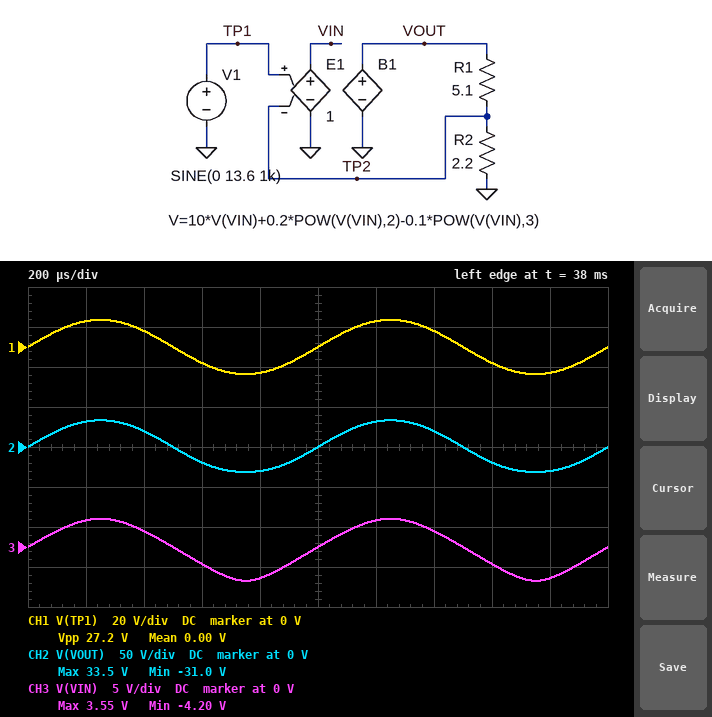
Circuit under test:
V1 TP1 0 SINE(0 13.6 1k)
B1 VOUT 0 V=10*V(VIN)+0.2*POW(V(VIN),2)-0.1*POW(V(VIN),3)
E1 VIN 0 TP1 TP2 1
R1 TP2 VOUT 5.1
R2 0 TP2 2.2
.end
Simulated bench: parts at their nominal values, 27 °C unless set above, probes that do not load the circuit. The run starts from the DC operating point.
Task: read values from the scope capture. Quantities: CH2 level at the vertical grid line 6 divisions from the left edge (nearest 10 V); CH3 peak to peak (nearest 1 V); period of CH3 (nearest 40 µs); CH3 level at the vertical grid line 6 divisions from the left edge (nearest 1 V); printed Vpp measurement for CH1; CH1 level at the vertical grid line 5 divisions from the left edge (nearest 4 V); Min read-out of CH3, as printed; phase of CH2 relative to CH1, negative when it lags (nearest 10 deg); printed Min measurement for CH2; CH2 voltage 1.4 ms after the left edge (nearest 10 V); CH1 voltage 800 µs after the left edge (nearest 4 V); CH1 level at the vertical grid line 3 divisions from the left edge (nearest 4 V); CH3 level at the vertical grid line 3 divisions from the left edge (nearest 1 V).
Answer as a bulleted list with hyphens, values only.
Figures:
- 30 V
- 8 V
- 1.00 ms
- 3 V
- 27.2 V
- 0 V
- -4.20 V
- 0 deg
- -31.0 V
- 20 V
- -12 V
- -8 V
- -2 V
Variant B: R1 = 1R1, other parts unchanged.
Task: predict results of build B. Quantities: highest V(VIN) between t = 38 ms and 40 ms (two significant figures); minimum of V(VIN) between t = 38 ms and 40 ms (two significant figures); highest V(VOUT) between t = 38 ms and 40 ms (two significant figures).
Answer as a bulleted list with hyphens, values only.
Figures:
- 1.8 V
- -1.9 V
- 18 V
